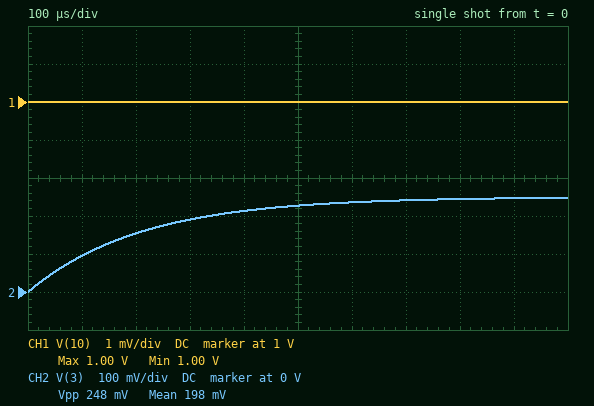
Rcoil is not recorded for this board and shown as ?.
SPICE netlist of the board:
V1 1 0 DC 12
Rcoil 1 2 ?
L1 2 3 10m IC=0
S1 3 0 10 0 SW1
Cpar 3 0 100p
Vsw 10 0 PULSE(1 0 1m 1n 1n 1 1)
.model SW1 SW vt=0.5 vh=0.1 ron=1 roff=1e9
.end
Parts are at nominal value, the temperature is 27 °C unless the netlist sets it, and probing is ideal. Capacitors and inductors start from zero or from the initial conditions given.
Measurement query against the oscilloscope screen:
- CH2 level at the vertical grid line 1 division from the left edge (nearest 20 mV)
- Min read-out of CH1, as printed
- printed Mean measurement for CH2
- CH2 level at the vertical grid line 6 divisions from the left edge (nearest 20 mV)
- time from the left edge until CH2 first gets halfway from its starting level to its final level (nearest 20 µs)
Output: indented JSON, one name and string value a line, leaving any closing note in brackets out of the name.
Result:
{
  "CH2 level at the vertical grid line 1 division from the left edge": "100 mV",
  "Min read-out of CH1, as printed": "1.00 V",
  "printed Mean measurement for CH2": "198 mV",
  "CH2 level at the vertical grid line 6 divisions from the left edge": "240 mV",
  "time from the left edge until CH2 first gets halfway from its starting level to its final level": "140 µs"
}
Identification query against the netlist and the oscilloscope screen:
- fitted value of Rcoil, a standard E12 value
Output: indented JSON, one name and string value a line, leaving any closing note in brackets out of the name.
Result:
{
  "fitted value of Rcoil, a standard E12 value": "47 Ω"
}
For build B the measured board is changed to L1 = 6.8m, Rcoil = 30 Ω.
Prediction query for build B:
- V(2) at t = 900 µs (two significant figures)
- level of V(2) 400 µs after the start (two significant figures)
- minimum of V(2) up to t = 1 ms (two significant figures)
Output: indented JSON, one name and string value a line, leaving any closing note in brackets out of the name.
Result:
{
  "V(2) at t = 900 µs": "580 mV",
  "level of V(2) 400 µs after the start": "2.3 V",
  "minimum of V(2) up to t = 1 ms": "510 mV"
}
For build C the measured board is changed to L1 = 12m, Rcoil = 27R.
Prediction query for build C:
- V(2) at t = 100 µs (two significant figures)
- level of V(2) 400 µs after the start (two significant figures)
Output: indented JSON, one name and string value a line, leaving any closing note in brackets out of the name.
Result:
{
  "V(2) at t = 100 µs": "9.6 V",
  "level of V(2) 400 µs after the start": "5.0 V"
}
